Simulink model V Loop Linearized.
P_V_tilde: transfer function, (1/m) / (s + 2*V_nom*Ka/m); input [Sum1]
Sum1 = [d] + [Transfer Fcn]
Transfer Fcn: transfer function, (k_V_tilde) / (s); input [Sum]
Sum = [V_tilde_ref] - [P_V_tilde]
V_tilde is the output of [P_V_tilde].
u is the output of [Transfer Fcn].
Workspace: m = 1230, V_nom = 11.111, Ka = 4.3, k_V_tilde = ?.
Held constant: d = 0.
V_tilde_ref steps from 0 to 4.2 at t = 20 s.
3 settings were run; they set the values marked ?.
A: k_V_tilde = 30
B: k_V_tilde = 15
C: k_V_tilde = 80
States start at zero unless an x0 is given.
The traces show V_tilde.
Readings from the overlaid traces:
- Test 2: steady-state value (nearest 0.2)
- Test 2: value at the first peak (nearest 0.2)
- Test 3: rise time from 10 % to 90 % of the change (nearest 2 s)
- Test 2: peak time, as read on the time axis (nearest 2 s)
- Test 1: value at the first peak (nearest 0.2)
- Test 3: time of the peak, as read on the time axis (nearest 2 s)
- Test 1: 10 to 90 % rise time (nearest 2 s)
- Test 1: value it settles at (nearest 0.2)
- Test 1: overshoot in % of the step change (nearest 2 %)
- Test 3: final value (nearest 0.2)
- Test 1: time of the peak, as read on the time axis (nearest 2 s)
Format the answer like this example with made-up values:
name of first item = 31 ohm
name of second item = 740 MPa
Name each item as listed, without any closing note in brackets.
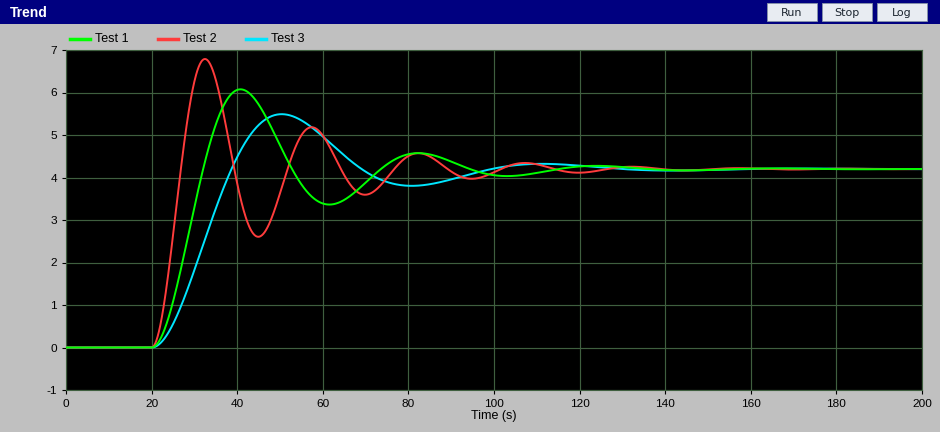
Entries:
Test 2: steady-state value = 4.2
Test 2: value at the first peak = 6.8
Test 3: rise time from 10 % to 90 % of the change = 12 s
Test 2: peak time, as read on the time axis = 32 s
Test 1: value at the first peak = 6.0
Test 3: time of the peak, as read on the time axis = 50 s
Test 1: 10 to 90 % rise time = 8 s
Test 1: value it settles at = 4.2
Test 1: overshoot in % of the step change = 44 %
Test 3: final value = 4.2
Test 1: time of the peak, as read on the time axis = 40 s
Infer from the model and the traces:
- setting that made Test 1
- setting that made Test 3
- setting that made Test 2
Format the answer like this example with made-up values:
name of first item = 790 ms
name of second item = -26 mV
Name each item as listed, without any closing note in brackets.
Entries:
setting that made Test 1 = A
setting that made Test 3 = B
setting that made Test 2 = C
